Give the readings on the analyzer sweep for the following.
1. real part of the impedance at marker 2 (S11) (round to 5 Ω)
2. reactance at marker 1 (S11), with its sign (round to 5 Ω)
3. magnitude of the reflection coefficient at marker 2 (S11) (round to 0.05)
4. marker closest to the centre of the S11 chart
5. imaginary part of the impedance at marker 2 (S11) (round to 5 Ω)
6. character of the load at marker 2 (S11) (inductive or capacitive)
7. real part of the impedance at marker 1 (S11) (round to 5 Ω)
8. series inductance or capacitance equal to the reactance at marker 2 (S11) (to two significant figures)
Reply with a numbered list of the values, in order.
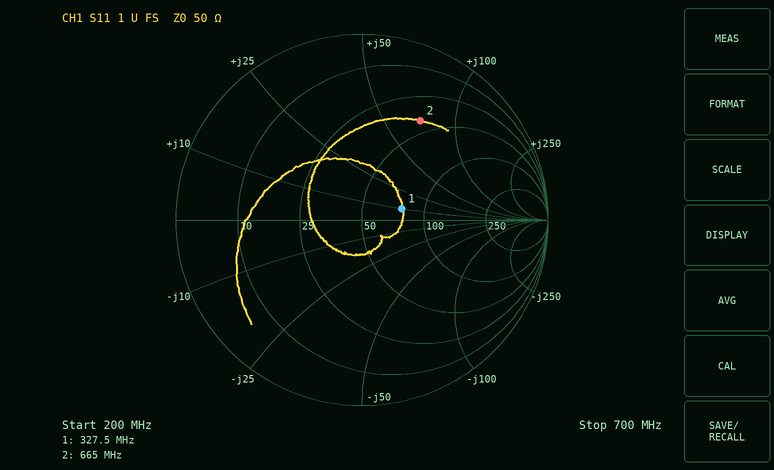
1. 40 Ω
2. +10 Ω
3. 0.60
4. marker 1
5. +70 Ω
6. inductive
7. 75 Ω
8. 17 nH
